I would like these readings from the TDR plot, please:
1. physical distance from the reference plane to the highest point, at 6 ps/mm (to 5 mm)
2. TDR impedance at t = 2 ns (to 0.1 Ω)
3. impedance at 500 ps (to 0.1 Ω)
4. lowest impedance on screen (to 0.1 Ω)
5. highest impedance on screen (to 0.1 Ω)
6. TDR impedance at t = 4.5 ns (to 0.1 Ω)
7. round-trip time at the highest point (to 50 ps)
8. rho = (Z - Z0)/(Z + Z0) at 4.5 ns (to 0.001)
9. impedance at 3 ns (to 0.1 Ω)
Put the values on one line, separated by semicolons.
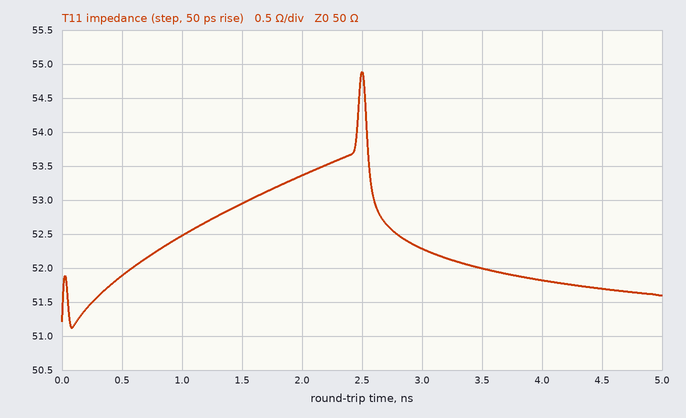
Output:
210 mm; 53.4 Ω; 51.9 Ω; 51.1 Ω; 54.9 Ω; 51.7 Ω; 2.50 ns; +0.017; 52.3 Ω
